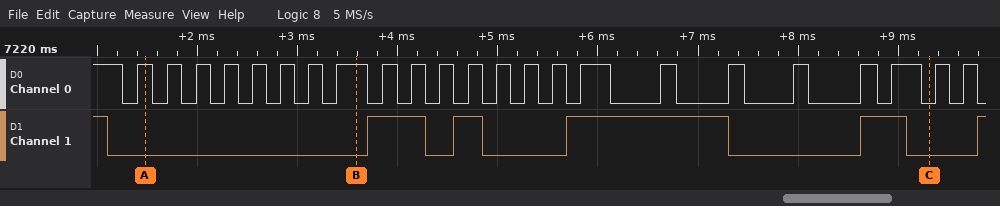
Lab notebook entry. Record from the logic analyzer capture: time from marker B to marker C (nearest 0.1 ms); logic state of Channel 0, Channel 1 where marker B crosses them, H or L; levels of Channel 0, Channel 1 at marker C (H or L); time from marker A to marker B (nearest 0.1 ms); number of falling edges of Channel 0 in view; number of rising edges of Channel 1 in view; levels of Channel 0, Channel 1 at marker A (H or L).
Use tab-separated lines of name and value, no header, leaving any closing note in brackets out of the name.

time from marker B to marker C	5.7 ms
logic state of Channel 0, Channel 1 where marker B crosses them, H or L	Channel 0=H, Channel 1=L
levels of Channel 0, Channel 1 at marker C	Channel 0=L, Channel 1=L
time from marker A to marker B	2.1 ms
number of falling edges of Channel 0 in view	24
number of rising edges of Channel 1 in view	5
levels of Channel 0, Channel 1 at marker A	Channel 0=H, Channel 1=L
